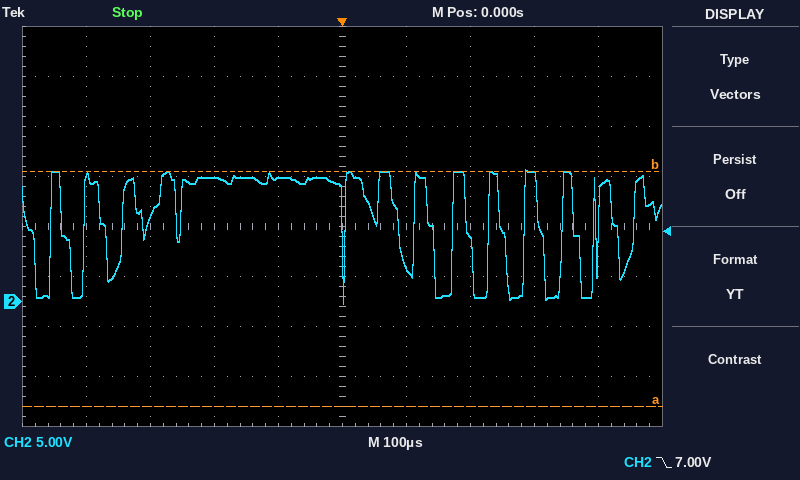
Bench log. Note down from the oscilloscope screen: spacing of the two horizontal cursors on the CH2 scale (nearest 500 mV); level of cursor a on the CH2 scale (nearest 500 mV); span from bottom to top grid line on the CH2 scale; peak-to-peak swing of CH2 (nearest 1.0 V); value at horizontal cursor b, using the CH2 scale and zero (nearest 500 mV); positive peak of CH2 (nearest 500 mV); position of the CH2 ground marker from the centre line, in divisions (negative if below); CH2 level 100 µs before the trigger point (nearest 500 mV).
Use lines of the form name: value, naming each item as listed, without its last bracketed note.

spacing of the two horizontal cursors on the CH2 scale: 23.5 V
level of cursor a on the CH2 scale: -10.5 V
span from bottom to top grid line on the CH2 scale: 40 V
peak-to-peak swing of CH2: 13.0 V
value at horizontal cursor b, using the CH2 scale and zero: 13.0 V
positive peak of CH2: 13.0 V
position of the CH2 ground marker from the centre line, in divisions: -1.5 div
CH2 level 100 µs before the trigger point: 12.5 V
